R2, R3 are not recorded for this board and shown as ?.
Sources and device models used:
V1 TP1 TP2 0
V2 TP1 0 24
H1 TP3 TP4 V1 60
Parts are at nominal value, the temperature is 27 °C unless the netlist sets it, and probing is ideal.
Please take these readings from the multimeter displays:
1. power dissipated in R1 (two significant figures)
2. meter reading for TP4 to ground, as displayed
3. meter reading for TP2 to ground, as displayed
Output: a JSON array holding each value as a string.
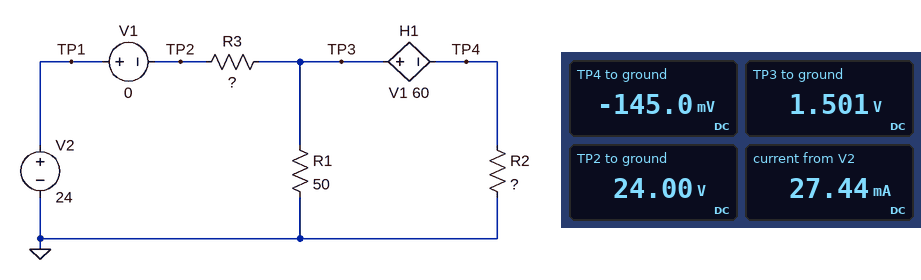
["45 mW", "-145.0 mV", "24.00 V"]
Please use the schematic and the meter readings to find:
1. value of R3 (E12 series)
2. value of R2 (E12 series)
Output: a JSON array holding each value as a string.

["820 Ω", "56 Ω"]
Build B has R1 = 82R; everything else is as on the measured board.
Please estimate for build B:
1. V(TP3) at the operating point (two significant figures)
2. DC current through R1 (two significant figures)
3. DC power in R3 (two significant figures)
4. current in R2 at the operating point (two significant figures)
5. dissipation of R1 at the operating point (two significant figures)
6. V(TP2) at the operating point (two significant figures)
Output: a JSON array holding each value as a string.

["1.9 V", "23 mA", "600 mW", "4.3 mA", "42 mW", "24 V"]
